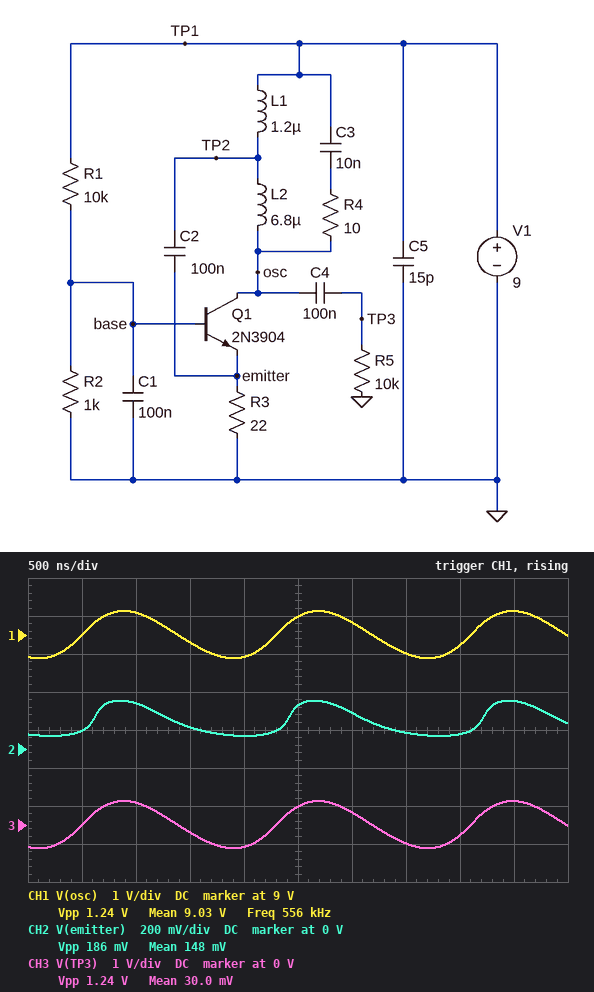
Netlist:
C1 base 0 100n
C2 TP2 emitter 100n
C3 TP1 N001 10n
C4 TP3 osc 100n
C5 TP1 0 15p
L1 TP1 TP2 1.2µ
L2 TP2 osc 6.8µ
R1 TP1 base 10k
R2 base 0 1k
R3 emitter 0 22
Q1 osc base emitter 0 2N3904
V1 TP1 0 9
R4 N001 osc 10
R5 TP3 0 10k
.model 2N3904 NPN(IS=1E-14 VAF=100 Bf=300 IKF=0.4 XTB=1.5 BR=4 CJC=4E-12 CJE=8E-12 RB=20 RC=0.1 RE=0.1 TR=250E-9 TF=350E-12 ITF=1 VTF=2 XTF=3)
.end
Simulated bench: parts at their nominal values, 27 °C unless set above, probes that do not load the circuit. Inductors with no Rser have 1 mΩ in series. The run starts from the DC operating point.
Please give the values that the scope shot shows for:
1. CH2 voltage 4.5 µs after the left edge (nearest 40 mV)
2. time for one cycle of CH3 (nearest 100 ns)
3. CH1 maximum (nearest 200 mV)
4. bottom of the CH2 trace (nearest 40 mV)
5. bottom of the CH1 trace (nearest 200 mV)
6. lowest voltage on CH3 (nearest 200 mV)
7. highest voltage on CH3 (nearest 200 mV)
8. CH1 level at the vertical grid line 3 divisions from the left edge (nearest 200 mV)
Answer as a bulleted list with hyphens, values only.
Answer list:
- 240 mV
- 1.8 µs
- 9.6 V
- 80 mV
- 8.4 V
- -600 mV
- 600 mV
- 8.8 V
